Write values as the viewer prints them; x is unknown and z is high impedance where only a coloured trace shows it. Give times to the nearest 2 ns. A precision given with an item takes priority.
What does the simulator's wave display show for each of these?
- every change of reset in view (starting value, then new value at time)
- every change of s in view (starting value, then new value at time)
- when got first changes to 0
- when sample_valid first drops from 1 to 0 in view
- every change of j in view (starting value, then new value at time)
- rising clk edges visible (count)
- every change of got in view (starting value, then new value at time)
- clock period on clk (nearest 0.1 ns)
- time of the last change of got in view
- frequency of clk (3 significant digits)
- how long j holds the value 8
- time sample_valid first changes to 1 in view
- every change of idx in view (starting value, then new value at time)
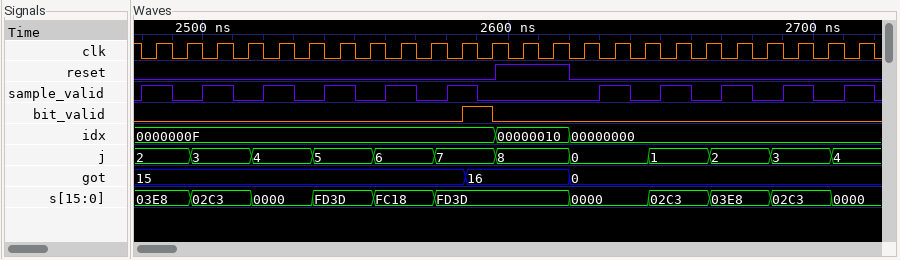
0, 1 at 2596 ns, 0 at 2620 ns
03E8, 02C3 at 2496 ns, 0000 at 2516 ns, FD3D at 2536 ns, FC18 at 2556 ns, FD3D at 2576 ns, 0000 at 2620 ns, 02C3 at 2646 ns, 03E8 at 2666 ns, 02C3 at 2686 ns, 0000 at 2706 ns
2620 ns
2490 ns
2, 3 at 2496 ns, 4 at 2516 ns, 5 at 2536 ns, 6 at 2556 ns, 7 at 2576 ns, 8 at 2596 ns, 0 at 2620 ns, 1 at 2646 ns, 2 at 2666 ns, 3 at 2686 ns, 4 at 2706 ns
24
15, 16 at 2586 ns, 0 at 2620 ns
10 ns
2620 ns
100 MHz
24 ns
2480 ns
0000000F, 00000010 at 2596 ns, 00000000 at 2620 ns
